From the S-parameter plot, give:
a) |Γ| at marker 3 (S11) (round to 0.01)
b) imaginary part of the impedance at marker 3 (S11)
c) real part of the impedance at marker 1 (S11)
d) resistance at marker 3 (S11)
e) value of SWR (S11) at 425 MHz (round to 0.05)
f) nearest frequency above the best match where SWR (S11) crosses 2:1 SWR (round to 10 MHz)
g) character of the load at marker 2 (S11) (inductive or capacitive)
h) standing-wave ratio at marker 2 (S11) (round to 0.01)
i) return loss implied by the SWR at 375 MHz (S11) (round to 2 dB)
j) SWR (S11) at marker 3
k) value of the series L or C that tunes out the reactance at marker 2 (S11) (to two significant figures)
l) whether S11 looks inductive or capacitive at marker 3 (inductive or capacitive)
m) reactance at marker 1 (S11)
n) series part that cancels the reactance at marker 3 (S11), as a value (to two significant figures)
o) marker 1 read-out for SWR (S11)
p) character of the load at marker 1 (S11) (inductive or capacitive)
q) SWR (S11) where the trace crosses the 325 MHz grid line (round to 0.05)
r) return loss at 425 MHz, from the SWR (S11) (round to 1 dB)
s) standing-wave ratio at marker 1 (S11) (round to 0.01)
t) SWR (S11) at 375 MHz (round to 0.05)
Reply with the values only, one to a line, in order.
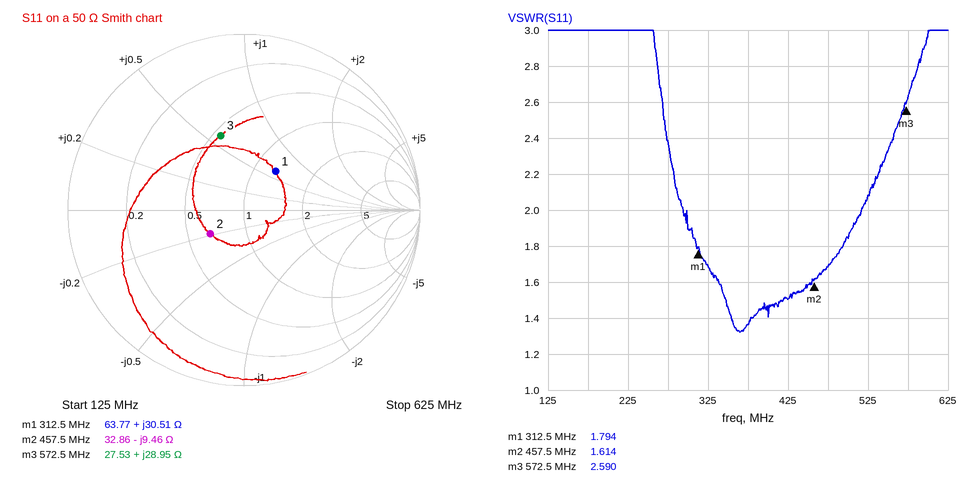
0.44
+28.95 Ω
63.77 Ω
27.53 Ω
1.50
520 MHz
capacitive
1.61
16 dB
2.590
3.3 nH
inductive
+30.51 Ω
9.6 pF
1.794
inductive
1.70
14 dB
1.79
1.35
